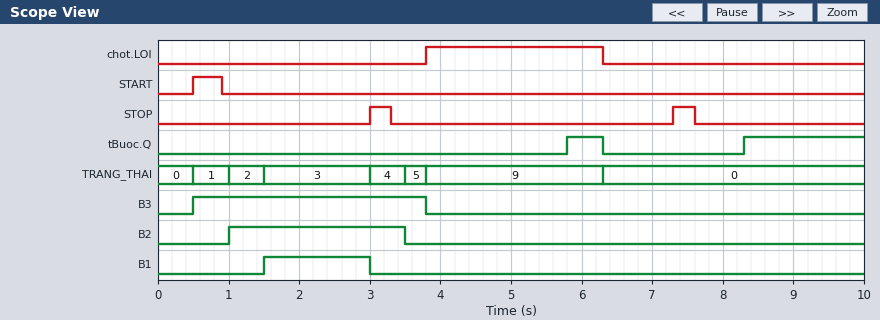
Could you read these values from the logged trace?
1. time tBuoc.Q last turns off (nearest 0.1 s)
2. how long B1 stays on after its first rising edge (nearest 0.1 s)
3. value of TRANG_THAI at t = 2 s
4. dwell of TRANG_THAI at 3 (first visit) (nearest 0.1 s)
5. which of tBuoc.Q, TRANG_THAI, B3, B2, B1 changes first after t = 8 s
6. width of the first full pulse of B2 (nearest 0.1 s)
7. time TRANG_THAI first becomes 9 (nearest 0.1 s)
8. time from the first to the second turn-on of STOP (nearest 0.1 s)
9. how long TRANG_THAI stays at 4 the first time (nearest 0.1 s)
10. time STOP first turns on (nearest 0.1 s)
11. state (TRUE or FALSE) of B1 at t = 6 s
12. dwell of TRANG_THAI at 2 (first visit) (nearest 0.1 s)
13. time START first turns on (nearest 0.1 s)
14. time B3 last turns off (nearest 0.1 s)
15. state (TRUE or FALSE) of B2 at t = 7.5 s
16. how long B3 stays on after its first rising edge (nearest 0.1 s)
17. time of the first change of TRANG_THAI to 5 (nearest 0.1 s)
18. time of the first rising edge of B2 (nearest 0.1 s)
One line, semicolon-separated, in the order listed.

6.3 s; 1.5 s; 3; 1.5 s; tBuoc.Q; 2.5 s; 3.8 s; 4.3 s; 0.5 s; 3.0 s; FALSE; 0.5 s; 0.5 s; 3.8 s; FALSE; 3.3 s; 3.5 s; 1.0 s
